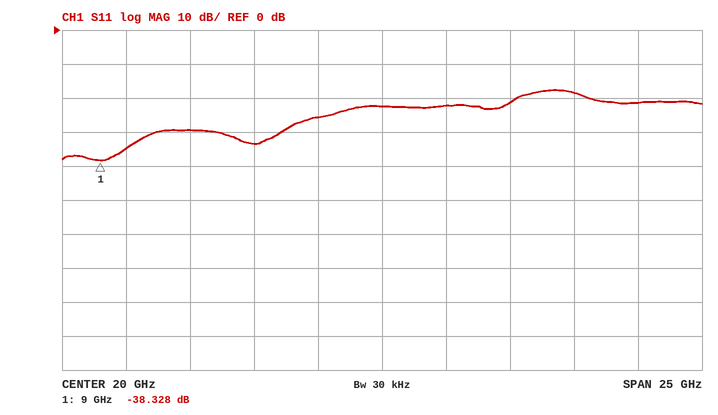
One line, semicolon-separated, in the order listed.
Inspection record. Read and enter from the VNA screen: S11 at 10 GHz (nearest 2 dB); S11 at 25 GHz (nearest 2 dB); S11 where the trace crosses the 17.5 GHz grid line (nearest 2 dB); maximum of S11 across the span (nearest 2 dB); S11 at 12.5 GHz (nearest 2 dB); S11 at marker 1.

-34 dB; -22 dB; -26 dB; -18 dB; -30 dB; -38.328 dB
